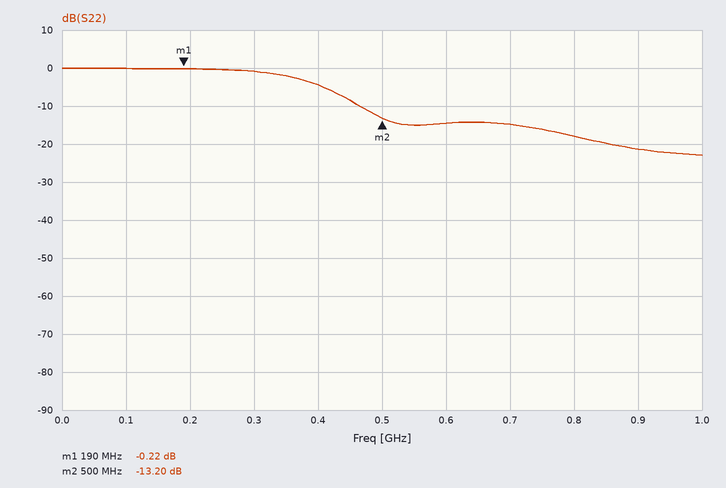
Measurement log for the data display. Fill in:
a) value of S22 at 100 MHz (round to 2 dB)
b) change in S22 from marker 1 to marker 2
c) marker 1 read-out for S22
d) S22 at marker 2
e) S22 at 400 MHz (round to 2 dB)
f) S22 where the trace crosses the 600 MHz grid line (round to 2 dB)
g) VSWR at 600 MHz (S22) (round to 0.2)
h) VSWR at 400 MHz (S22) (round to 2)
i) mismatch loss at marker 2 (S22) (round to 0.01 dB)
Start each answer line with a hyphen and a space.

- 0 dB
- -12.98 dB
- -0.22 dB
- -13.20 dB
- -4 dB
- -14 dB
- 1.4
- 4
- 0.21 dB
